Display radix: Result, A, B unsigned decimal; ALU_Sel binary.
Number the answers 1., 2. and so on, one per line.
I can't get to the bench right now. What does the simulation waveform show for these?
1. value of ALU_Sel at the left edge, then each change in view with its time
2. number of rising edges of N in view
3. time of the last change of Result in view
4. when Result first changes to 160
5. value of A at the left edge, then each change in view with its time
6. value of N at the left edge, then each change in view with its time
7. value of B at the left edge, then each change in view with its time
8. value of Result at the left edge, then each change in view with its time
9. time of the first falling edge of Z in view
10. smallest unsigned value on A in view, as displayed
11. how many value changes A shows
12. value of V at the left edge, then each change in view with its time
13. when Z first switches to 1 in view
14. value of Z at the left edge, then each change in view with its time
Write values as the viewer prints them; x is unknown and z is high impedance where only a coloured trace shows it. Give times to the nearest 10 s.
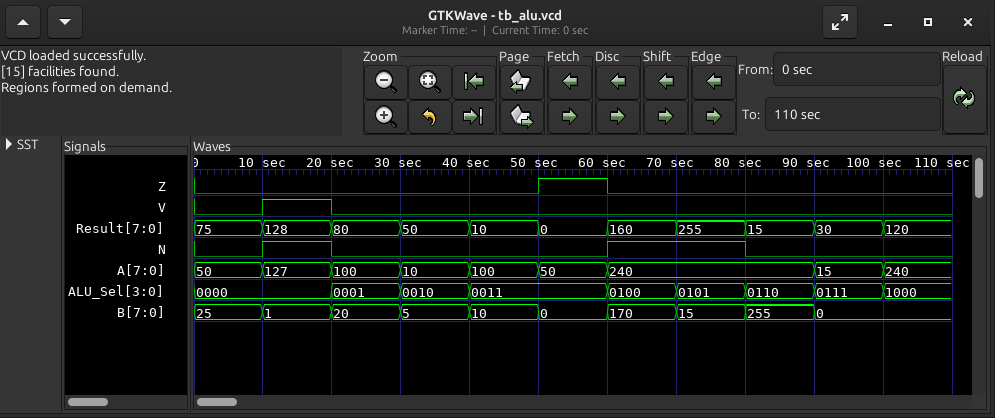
1. 0000, 0001 at 20 s, 0010 at 30 s, 0011 at 40 s, 0100 at 60 s, 0101 at 70 s, 0110 at 80 s, 0111 at 90 s, 1000 at 100 s
2. 2
3. 100 s
4. 60 s
5. 50, 127 at 10 s, 100 at 20 s, 10 at 30 s, 100 at 40 s, 50 at 50 s, 240 at 60 s, 15 at 90 s, 240 at 100 s
6. 0, 1 at 10 s, 0 at 20 s, 1 at 60 s, 0 at 80 s
7. 25, 1 at 10 s, 20 at 20 s, 5 at 30 s, 10 at 40 s, 0 at 50 s, 170 at 60 s, 15 at 70 s, 255 at 80 s, 0 at 90 s
8. 75, 128 at 10 s, 80 at 20 s, 50 at 30 s, 10 at 40 s, 0 at 50 s, 160 at 60 s, 255 at 70 s, 15 at 80 s, 30 at 90 s, 120 at 100 s
9. 60 s
10. 10
11. 8
12. 0, 1 at 10 s, 0 at 20 s
13. 50 s
14. 0, 1 at 50 s, 0 at 60 s
